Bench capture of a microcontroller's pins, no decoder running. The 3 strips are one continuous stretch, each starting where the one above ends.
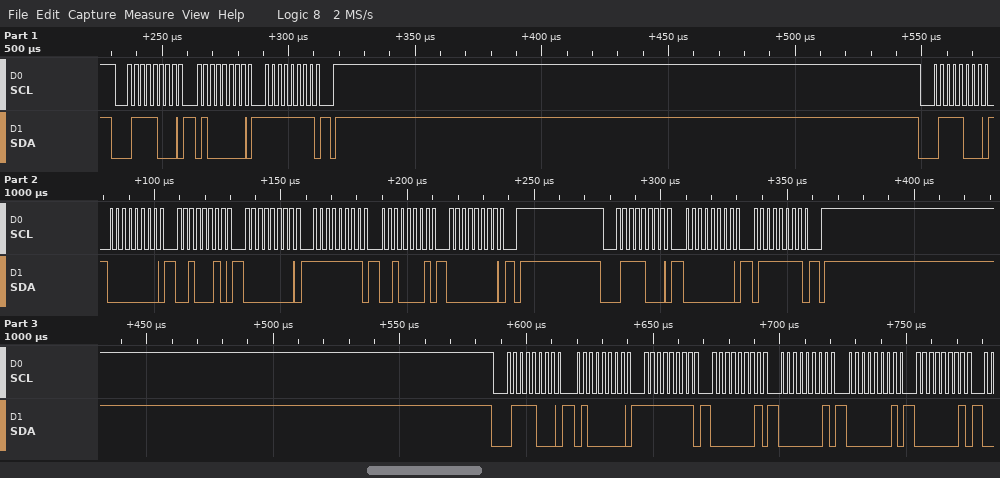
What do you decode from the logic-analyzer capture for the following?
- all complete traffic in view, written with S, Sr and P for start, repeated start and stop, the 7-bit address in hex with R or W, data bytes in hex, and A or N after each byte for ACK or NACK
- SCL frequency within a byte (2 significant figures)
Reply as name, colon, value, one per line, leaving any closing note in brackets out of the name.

all complete traffic in view, written with S, Sr and P for start, repeated start and stop, the 7-bit address in hex with R or W, data bytes in hex, and A or N after each byte for ACK or NACK: S 3CW A 40 A FF A P S 3CW A 00 A 22 A 00 A FF A 21 A 00 A P S 3CW A 00 A 7F A P S 3CW A 40 A FF A 01 A 01 A 01 A 01 A
SCL frequency within a byte: 400 kHz
